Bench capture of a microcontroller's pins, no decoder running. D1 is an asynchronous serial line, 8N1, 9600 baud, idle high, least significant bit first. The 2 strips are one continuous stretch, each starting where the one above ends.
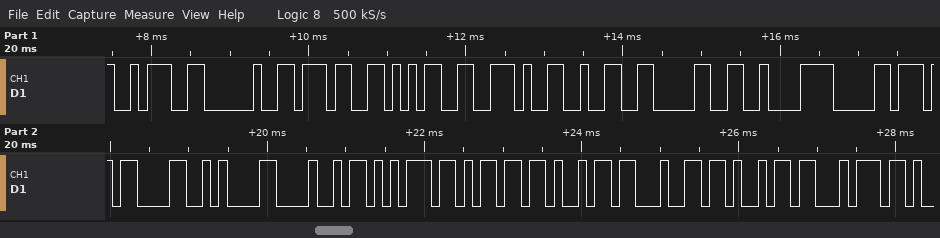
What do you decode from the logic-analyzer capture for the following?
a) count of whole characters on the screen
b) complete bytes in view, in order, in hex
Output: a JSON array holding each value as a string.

["18", "3A 20 37 35 2E 32 30 C2 B0 0D 0A 48 75 6D 69 64 69 74"]
